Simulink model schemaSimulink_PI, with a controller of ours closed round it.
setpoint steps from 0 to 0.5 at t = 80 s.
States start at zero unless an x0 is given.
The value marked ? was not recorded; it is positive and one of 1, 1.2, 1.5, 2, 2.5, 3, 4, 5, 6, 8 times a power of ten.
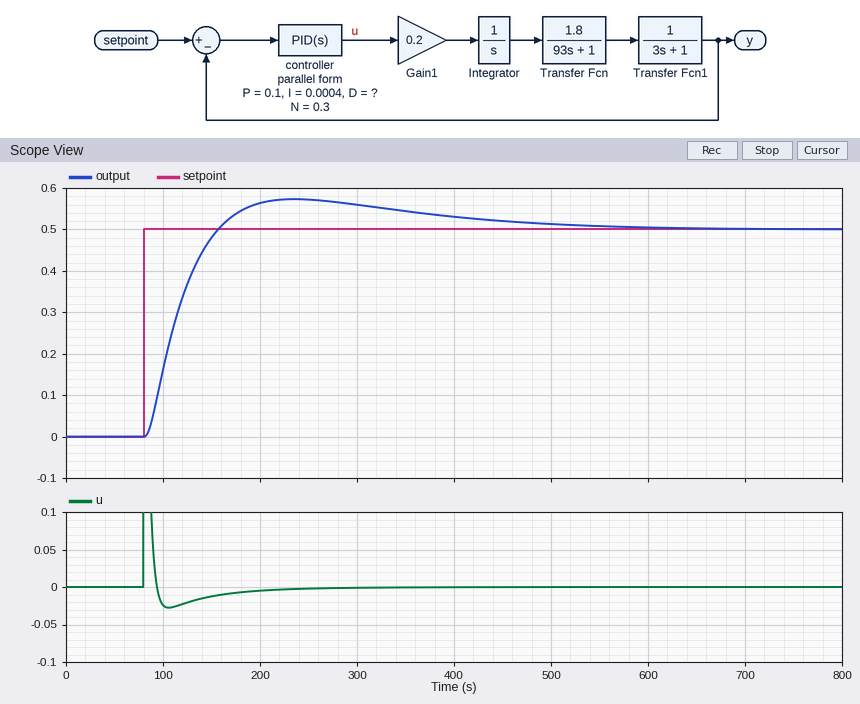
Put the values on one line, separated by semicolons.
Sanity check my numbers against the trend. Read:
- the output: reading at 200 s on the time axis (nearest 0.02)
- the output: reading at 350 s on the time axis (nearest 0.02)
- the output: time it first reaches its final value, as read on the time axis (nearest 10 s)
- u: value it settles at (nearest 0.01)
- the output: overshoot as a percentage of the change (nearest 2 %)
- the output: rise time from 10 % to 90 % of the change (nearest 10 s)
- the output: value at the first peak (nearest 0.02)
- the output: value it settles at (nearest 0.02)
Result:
0.56; 0.54; 160 s; 0.00; 14 %; 50 s; 0.58; 0.50
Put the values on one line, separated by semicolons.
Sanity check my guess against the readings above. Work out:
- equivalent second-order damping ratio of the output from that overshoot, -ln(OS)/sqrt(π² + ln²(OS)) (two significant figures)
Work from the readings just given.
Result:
0.53
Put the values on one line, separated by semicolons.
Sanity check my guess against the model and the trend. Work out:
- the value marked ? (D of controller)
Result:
6
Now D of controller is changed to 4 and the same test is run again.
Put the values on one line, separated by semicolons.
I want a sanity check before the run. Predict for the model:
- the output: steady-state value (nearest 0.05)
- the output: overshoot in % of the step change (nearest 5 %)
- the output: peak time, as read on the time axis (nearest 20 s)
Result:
0.50; 25 %; 240 s
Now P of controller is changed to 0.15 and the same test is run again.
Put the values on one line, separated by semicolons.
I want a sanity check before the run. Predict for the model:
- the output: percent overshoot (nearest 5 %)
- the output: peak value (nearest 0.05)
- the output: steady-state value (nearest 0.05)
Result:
20 %; 0.60; 0.50
